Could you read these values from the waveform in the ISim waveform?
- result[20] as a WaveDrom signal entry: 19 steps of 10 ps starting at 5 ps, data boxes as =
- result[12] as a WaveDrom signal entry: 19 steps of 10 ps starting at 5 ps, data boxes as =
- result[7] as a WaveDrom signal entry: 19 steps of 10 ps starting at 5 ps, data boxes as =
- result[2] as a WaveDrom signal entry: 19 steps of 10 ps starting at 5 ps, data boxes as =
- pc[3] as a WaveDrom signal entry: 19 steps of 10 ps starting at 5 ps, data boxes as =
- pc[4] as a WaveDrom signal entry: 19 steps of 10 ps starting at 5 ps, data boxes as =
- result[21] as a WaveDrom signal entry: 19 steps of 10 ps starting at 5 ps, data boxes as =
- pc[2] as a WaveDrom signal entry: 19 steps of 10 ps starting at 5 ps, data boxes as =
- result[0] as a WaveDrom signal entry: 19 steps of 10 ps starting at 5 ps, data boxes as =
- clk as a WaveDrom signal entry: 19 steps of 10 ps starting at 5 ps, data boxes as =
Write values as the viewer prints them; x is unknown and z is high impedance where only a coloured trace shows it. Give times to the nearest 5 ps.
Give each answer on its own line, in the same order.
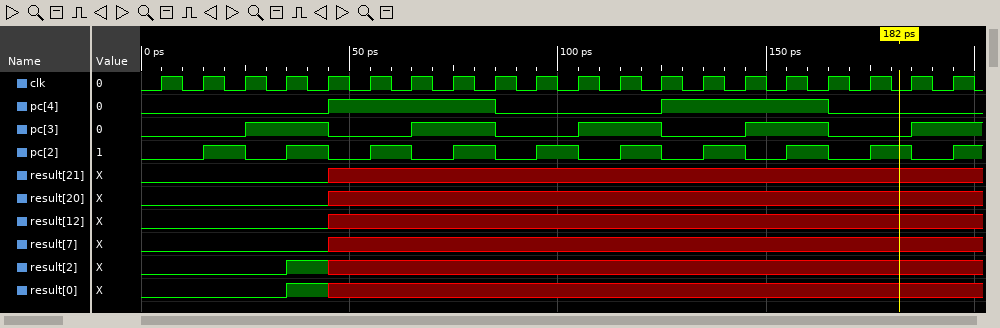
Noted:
{name: 'result[20]', wave: '0...x..............'}
{name: 'result[12]', wave: '0...x..............'}
{name: 'result[7]', wave: '0...x..............'}
{name: 'result[2]', wave: '0..1x..............'}
{name: 'pc[3]', wave: '0.1.0.1.0.1.0.1.0.1'}
{name: 'pc[4]', wave: '0...1...0...1...0..'}
{name: 'result[21]', wave: '0...x..............'}
{name: 'pc[2]', wave: '0101010101010101010'}
{name: 'result[0]', wave: '0..1x..............'}
{name: 'clk', wave: 'p..................'}
